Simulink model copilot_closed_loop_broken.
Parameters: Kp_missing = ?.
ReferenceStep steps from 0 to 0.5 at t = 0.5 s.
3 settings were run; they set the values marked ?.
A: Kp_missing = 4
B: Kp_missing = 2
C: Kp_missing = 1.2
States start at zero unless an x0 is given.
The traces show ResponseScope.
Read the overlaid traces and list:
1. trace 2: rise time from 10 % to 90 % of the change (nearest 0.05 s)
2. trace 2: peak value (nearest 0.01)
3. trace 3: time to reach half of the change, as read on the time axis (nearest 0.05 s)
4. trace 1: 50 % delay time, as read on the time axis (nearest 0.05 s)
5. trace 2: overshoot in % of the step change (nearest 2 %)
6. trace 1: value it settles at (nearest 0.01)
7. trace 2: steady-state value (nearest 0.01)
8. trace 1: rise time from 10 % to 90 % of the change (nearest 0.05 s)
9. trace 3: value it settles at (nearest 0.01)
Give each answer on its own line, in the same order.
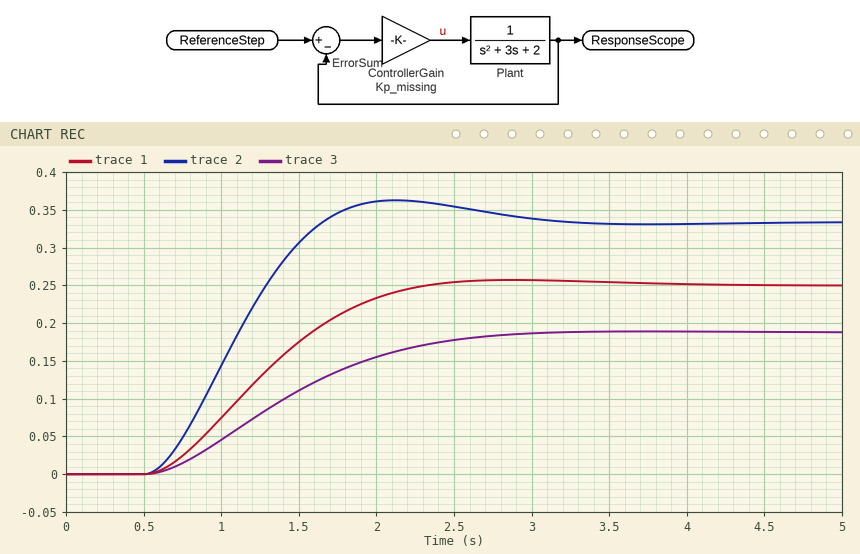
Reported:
0.75 s
0.36
1.35 s
1.25 s
8 %
0.25
0.33
1.15 s
0.19
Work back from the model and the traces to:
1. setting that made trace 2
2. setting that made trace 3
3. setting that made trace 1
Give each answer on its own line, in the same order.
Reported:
A
C
B
